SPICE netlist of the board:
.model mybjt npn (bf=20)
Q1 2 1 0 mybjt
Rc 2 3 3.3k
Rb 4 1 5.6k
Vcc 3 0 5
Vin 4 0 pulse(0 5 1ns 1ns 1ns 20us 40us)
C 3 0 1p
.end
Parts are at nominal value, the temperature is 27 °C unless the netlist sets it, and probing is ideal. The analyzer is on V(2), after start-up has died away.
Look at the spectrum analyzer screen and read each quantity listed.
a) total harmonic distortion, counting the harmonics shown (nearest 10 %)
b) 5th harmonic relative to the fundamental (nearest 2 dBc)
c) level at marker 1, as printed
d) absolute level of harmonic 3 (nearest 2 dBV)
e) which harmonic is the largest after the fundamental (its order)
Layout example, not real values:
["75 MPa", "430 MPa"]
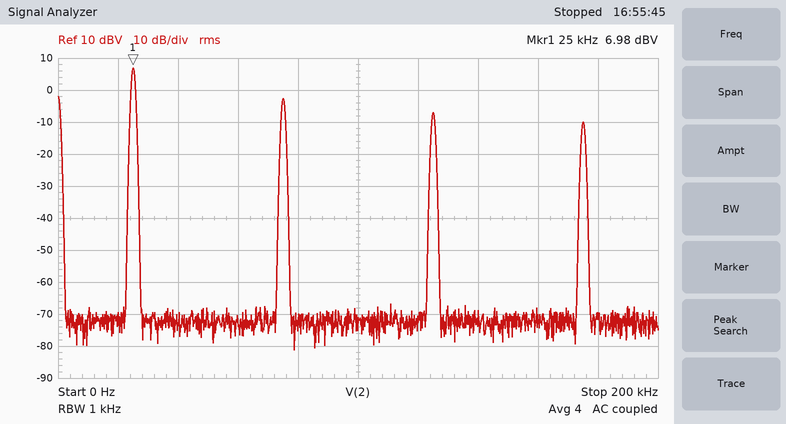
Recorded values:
["40 %", "-14 dBc", "6.98 dBV", "-2 dBV", "3"]
